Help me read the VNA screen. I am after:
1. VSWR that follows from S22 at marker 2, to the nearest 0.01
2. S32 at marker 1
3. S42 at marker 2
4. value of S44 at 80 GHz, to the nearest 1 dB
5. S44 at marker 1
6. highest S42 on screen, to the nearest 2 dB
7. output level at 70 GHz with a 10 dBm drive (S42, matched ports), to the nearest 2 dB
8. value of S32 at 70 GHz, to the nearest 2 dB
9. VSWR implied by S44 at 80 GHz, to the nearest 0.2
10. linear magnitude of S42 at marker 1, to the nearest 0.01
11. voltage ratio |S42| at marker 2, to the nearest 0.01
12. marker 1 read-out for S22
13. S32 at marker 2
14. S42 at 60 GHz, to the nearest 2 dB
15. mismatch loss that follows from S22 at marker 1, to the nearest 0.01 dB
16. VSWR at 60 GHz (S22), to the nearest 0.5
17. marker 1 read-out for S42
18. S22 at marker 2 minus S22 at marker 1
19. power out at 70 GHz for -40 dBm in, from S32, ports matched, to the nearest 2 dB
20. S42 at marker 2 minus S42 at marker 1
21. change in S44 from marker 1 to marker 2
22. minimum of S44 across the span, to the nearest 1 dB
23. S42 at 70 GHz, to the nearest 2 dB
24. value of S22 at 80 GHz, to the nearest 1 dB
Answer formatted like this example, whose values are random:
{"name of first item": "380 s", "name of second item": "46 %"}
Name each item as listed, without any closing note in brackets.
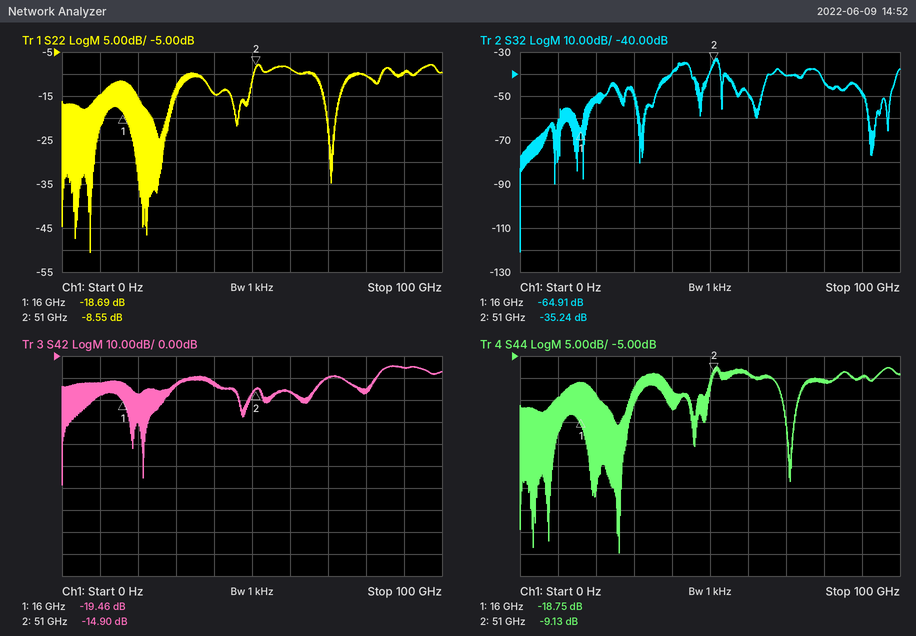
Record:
{"VSWR that follows from S22 at marker 2, to the nearest 0.01": "2.19", "S32 at marker 1": "-64.91 dB", "S42 at marker 2": "-14.90 dB", "value of S44 at 80 GHz, to the nearest 1 dB": "-11 dB", "S44 at marker 1": "-18.75 dB", "highest S42 on screen, to the nearest 2 dB": "-4 dB", "output level at 70 GHz with a 10 dBm drive (S42, matched ports), to the nearest 2 dB": "0 dBm", "value of S32 at 70 GHz, to the nearest 2 dB": "-40 dB", "VSWR implied by S44 at 80 GHz, to the nearest 0.2": "1.8", "linear magnitude of S42 at marker 1, to the nearest 0.01": "0.11", "voltage ratio |S42| at marker 2, to the nearest 0.01": "0.18", "marker 1 read-out for S22": "-18.69 dB", "S32 at marker 2": "-35.24 dB", "S42 at 60 GHz, to the nearest 2 dB": "-16 dB", "mismatch loss that follows from S22 at marker 1, to the nearest 0.01 dB": "0.06 dB", "VSWR at 60 GHz (S22), to the nearest 0.5": "2.0", "marker 1 read-out for S42": "-19.46 dB", "S22 at marker 2 minus S22 at marker 1": "10.14 dB", "power out at 70 GHz for -40 dBm in, from S32, ports matched, to the nearest 2 dB": "-80 dBm", "S42 at marker 2 minus S42 at marker 1": "4.56 dB", "change in S44 from marker 1 to marker 2": "9.62 dB", "minimum of S44 across the span, to the nearest 1 dB": "-50 dB", "S42 at 70 GHz, to the nearest 2 dB": "-10 dB", "value of S22 at 80 GHz, to the nearest 1 dB": "-10 dB"}
